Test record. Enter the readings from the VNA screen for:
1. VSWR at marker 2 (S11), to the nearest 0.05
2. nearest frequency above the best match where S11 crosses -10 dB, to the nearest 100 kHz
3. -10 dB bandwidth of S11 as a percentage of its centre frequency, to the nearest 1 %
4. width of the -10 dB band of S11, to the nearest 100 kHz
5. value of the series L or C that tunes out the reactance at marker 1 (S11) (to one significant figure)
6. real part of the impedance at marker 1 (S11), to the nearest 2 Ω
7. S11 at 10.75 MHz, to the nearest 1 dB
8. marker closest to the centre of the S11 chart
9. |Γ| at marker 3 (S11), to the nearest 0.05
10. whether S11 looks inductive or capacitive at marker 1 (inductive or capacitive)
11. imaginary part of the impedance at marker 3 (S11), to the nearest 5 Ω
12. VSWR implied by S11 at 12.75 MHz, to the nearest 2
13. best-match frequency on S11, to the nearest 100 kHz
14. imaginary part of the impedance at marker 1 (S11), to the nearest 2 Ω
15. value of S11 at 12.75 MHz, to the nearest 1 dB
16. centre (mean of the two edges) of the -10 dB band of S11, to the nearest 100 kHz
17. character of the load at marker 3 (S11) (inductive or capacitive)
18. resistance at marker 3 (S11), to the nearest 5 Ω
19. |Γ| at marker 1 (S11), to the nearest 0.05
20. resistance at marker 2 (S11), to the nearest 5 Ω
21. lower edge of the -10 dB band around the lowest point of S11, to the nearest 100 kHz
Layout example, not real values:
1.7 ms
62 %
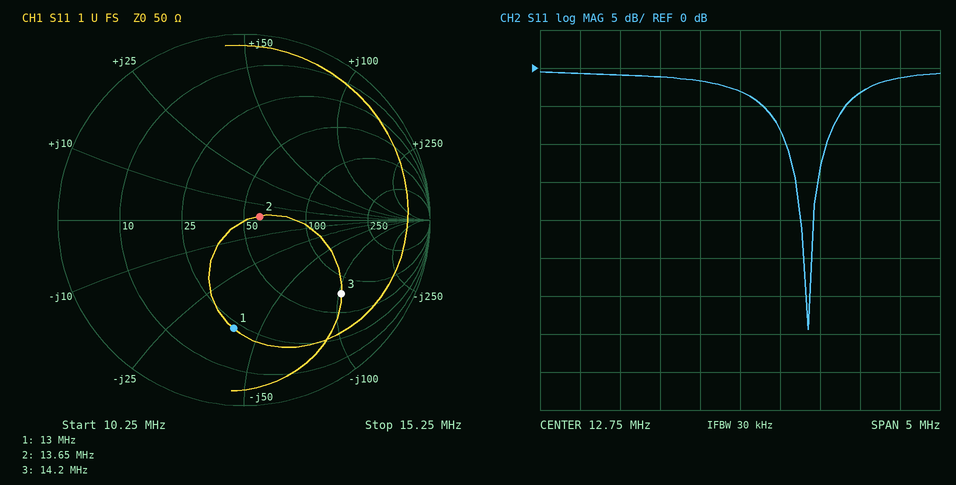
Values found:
1.20
13.8 MHz
4 %
500 kHz
500 nH
22 Ω
-1 dB
marker 2
0.65
capacitive
-105 Ω
6
13.6 MHz
-40 Ω
-3 dB
13.6 MHz
capacitive
75 Ω
0.60
60 Ω
13.3 MHz
